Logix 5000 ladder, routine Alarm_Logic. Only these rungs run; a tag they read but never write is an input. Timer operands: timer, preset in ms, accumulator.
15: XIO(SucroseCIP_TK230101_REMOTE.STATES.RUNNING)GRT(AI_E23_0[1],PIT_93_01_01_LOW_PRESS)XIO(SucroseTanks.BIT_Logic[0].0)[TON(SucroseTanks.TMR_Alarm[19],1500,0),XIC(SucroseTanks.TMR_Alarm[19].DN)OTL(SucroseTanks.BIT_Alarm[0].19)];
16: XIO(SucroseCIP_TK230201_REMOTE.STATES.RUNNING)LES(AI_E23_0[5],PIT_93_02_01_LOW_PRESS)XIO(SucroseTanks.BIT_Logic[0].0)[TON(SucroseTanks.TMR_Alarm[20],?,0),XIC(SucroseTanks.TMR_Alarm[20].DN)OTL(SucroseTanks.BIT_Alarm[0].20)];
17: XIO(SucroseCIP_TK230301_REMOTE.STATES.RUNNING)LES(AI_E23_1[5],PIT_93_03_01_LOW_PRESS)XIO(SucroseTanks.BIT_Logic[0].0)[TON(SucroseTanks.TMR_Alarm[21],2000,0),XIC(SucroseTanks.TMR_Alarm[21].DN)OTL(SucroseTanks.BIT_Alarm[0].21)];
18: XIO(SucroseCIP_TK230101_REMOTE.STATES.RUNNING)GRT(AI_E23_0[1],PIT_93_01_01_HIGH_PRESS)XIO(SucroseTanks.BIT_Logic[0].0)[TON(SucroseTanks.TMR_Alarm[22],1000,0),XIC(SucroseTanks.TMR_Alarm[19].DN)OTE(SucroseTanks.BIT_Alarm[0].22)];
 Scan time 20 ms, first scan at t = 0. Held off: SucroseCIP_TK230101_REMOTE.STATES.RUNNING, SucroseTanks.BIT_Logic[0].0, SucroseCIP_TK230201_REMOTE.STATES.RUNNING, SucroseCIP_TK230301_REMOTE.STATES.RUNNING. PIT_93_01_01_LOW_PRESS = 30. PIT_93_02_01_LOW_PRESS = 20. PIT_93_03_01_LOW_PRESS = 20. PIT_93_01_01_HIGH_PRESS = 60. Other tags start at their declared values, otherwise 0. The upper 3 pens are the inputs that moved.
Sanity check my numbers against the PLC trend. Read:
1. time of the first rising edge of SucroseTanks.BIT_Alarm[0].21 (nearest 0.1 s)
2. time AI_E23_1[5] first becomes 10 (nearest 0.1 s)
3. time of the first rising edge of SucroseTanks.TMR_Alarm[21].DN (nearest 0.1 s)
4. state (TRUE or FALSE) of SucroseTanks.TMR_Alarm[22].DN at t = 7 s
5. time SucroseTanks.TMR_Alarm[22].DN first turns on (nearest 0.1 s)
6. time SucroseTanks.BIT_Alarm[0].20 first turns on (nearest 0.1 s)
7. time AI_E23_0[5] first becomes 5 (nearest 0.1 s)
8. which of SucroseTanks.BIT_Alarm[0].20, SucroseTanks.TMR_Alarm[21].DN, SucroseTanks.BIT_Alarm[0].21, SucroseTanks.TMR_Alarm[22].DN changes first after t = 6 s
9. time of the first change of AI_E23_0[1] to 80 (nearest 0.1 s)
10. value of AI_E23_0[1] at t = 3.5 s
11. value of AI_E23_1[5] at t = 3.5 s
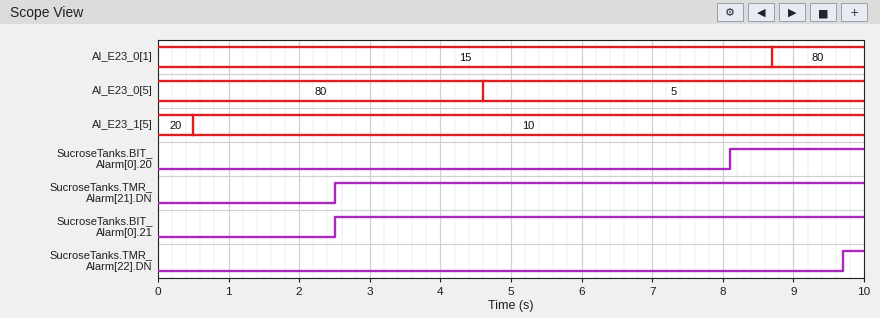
2.5 s
0.5 s
2.5 s
FALSE
9.7 s
8.1 s
4.6 s
SucroseTanks.BIT_Alarm[0].20
8.7 s
15
10
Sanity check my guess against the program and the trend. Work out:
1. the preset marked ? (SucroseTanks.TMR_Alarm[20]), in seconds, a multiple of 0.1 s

3.5 s
